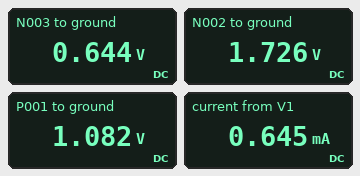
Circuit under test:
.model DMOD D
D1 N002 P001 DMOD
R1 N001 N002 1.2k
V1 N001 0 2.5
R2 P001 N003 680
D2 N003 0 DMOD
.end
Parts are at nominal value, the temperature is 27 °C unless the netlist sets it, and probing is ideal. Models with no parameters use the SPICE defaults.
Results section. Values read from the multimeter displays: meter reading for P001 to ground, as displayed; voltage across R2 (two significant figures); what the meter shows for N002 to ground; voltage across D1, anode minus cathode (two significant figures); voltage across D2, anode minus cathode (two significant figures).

1.082 V
440 mV
1.726 V
640 mV
640 mV
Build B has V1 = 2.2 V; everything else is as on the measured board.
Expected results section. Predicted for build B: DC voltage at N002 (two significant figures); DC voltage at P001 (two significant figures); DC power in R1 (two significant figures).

1.6 V
970 mV
290 µW
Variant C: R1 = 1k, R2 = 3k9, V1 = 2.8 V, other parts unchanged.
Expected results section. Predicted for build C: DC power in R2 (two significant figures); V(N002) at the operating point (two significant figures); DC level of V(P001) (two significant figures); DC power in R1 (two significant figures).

390 µW
2.5 V
1.9 V
100 µW
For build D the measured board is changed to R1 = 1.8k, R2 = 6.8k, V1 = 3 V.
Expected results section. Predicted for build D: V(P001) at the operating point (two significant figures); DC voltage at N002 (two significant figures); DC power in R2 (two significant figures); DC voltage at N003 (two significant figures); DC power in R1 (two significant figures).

2.0 V
2.6 V
290 µW
610 mV
76 µW
